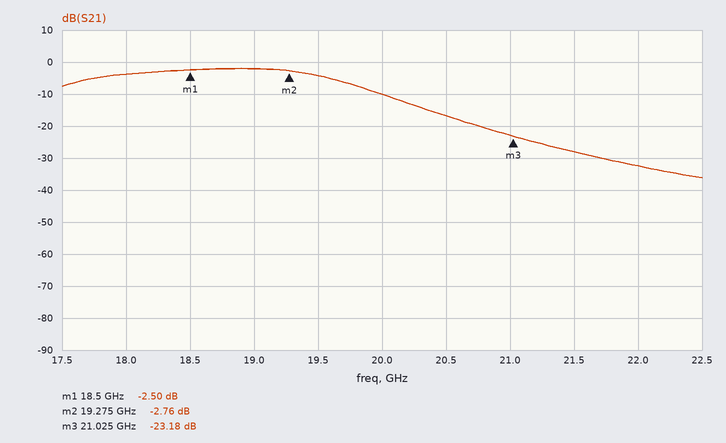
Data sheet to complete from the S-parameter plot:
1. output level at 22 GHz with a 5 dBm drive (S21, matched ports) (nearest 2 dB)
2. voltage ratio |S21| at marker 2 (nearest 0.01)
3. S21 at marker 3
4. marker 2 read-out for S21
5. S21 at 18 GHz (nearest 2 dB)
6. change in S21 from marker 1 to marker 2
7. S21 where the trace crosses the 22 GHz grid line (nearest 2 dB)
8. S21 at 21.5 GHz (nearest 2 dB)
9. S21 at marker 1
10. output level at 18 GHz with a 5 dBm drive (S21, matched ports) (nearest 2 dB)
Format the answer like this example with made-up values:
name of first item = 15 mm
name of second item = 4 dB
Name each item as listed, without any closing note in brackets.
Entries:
output level at 22 GHz with a 5 dBm drive (S21, matched ports) = -28 dBm
voltage ratio |S21| at marker 2 = 0.73
S21 at marker 3 = -23.18 dB
marker 2 read-out for S21 = -2.76 dB
S21 at 18 GHz = -4 dB
change in S21 from marker 1 to marker 2 = -0.26 dB
S21 where the trace crosses the 22 GHz grid line = -32 dB
S21 at 21.5 GHz = -28 dB
S21 at marker 1 = -2.50 dB
output level at 18 GHz with a 5 dBm drive (S21, matched ports) = 2 dBm
